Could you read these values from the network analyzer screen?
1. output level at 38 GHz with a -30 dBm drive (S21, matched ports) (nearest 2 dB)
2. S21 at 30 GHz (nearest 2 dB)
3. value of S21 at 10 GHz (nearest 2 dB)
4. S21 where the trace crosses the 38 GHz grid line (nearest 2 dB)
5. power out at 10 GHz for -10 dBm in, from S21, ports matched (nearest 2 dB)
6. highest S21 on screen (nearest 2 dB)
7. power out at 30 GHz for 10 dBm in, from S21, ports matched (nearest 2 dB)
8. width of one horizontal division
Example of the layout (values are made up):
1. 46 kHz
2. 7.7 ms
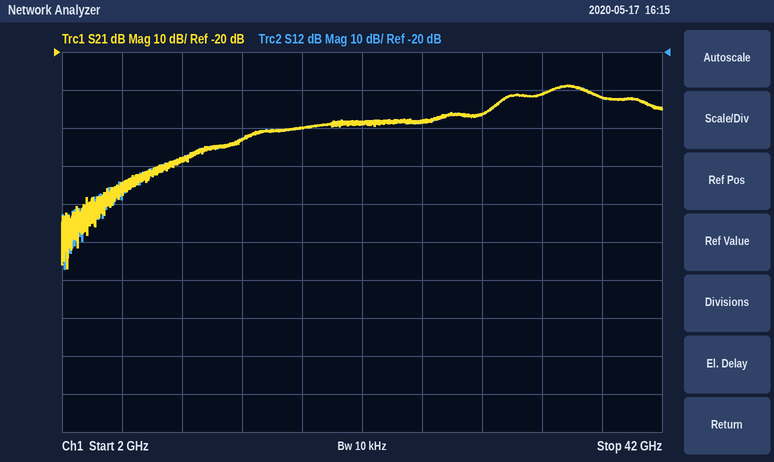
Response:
1. -62 dBm
2. -36 dB
3. -48 dB
4. -32 dB
5. -58 dBm
6. -28 dB
7. -26 dBm
8. 4 GHz
